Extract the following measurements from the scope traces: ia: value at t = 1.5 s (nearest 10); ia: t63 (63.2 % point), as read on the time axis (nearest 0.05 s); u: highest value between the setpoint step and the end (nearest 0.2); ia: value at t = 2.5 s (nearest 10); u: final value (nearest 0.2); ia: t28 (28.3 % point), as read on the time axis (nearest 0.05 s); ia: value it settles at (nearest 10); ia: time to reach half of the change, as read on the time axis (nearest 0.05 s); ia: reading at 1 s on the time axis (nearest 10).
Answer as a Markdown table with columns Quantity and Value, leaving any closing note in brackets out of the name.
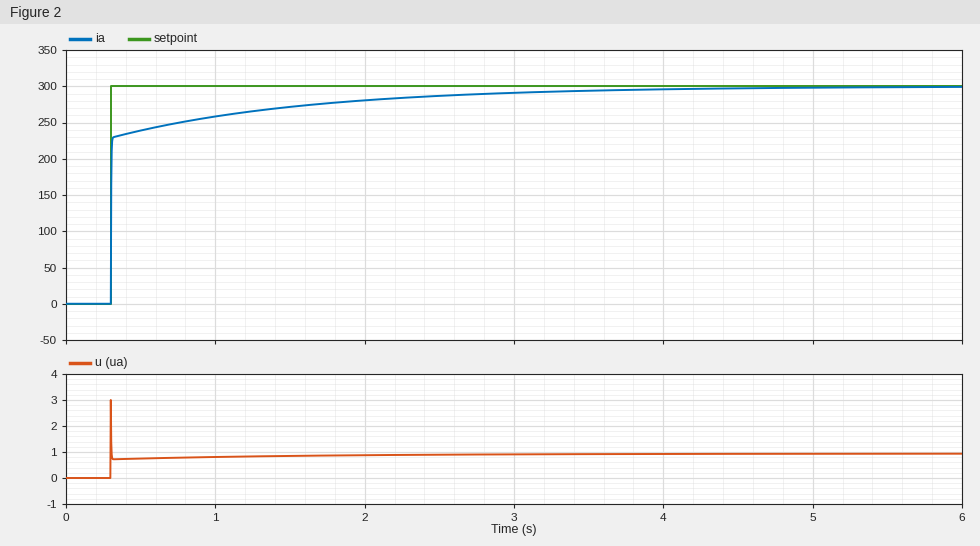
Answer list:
| Quantity | Value |
|---|---|
| ia: value at t = 1.5 s | 270 |
| ia: t63 (63.2 % point), as read on the time axis | 0.30 s |
| u: highest value between the setpoint step and the end | 3.0 |
| ia: value at t = 2.5 s | 290 |
| u: final value | 1.0 |
| ia: t28 (28.3 % point), as read on the time axis | 0.30 s |
| ia: value it settles at | 300 |
| ia: time to reach half of the change, as read on the time axis | 0.30 s |
| ia: reading at 1 s on the time axis | 260 |
